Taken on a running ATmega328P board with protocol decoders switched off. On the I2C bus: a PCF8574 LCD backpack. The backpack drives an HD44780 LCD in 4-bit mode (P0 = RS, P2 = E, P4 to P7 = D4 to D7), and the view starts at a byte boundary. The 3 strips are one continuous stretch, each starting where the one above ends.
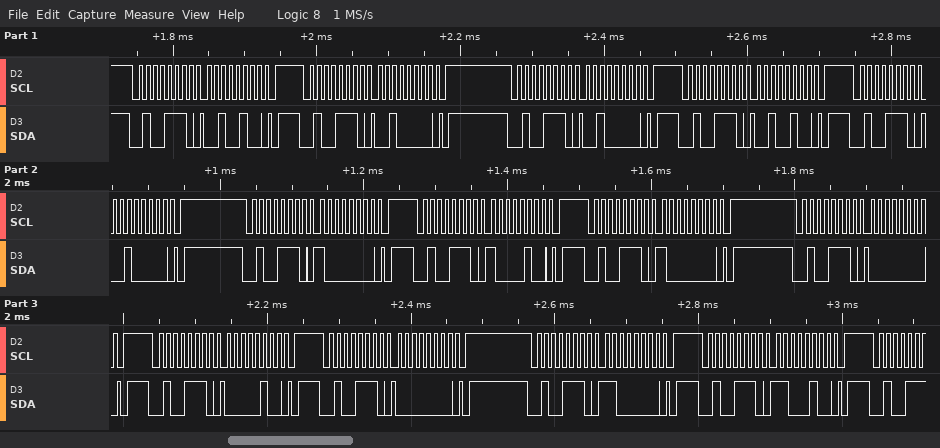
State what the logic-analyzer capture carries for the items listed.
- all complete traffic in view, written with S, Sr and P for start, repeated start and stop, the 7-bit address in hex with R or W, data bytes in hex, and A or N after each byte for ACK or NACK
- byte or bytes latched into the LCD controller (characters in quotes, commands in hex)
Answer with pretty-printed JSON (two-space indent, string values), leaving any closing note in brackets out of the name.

{
  "all complete traffic in view, written with S, Sr and P for start, repeated start and stop, the 7-bit address in hex with R or W, data bytes in hex, and A or N after each byte for ACK or NACK": "S 27W A 24 A P S 27W A 20 A P S 27W A 20 A P S 27W A 24 A P S 27W A 20 A P S 27W A 80 A P S 27W A 84 A P S 27W A 80 A P S 27W A 00 A P S 27W A 04 A P S 27W A 00 A P S 27W A C0 A P S 27W A C4 A P",
  "byte or bytes latched into the LCD controller": "0x28"
}
